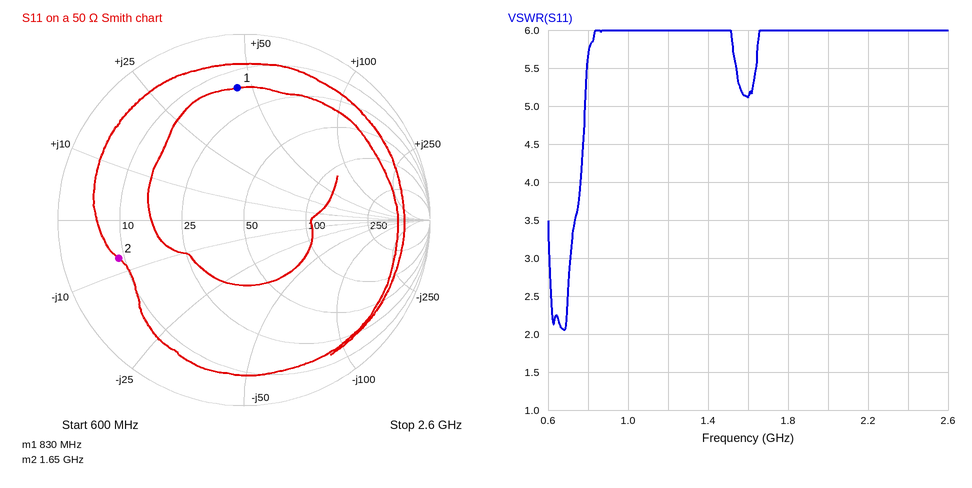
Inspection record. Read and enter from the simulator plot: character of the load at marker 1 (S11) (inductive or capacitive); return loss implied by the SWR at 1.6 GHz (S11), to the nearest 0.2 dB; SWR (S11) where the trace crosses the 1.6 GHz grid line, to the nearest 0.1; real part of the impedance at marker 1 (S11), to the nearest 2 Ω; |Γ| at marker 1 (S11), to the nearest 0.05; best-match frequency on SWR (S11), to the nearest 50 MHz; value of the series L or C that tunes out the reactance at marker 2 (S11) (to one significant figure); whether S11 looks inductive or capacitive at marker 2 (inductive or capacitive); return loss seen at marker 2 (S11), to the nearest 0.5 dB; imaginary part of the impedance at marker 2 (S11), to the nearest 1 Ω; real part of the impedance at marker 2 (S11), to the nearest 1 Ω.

inductive
3.4 dB
5.1
16 Ω
0.70
700 MHz
700 pH
capacitive
3.0 dB
-7 Ω
9 Ω
